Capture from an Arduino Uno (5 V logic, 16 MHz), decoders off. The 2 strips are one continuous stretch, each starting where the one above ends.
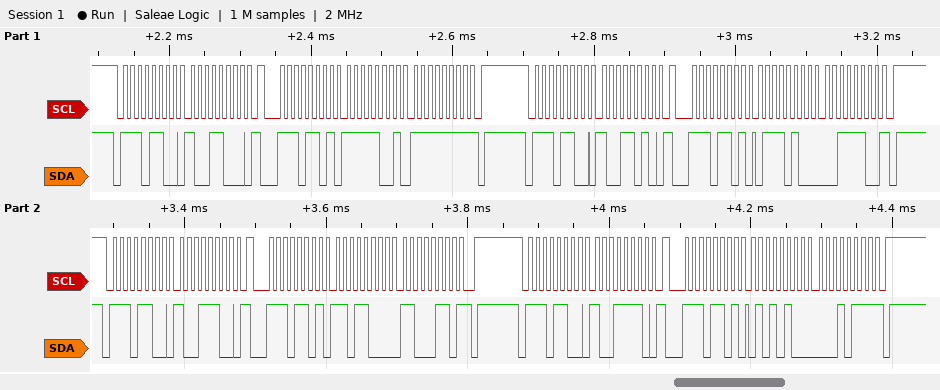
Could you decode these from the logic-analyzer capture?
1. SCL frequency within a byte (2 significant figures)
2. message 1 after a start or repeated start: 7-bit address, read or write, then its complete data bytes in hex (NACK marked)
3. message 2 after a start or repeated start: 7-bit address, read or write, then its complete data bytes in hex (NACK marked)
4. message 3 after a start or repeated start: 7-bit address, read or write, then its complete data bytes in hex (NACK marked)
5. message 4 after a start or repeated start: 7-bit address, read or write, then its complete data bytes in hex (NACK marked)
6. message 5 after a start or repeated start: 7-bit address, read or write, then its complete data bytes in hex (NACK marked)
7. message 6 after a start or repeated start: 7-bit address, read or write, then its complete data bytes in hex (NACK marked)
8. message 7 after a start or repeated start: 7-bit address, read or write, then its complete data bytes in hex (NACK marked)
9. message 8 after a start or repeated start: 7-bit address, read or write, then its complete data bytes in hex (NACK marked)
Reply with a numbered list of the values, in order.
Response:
1. 100 kHz
2. 0x76 write: 98
3. 0x76 read: F9 FF NACK
4. 0x76 write: 9A
5. 0x76 read: 74 3C NACK
6. 0x76 write: 9C
7. 0x76 read: D8 C6 NACK
8. 0x76 write: 9E
9. 0x76 read: 54 17 NACK
